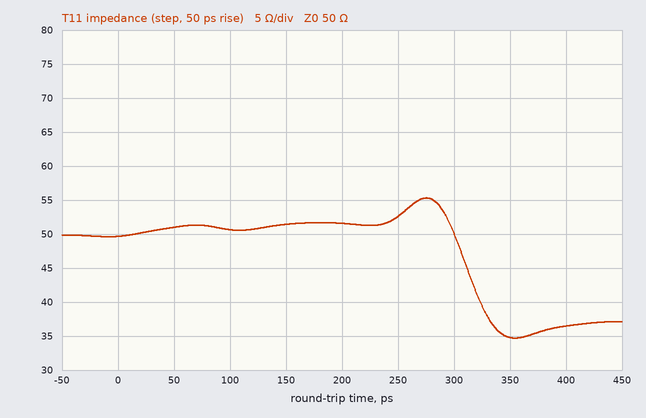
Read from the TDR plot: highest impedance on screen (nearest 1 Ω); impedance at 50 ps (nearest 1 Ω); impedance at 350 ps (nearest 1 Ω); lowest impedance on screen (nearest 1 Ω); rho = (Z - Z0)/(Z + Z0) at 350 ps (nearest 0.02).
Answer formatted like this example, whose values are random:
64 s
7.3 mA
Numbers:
55 Ω
51 Ω
35 Ω
35 Ω
-0.18
